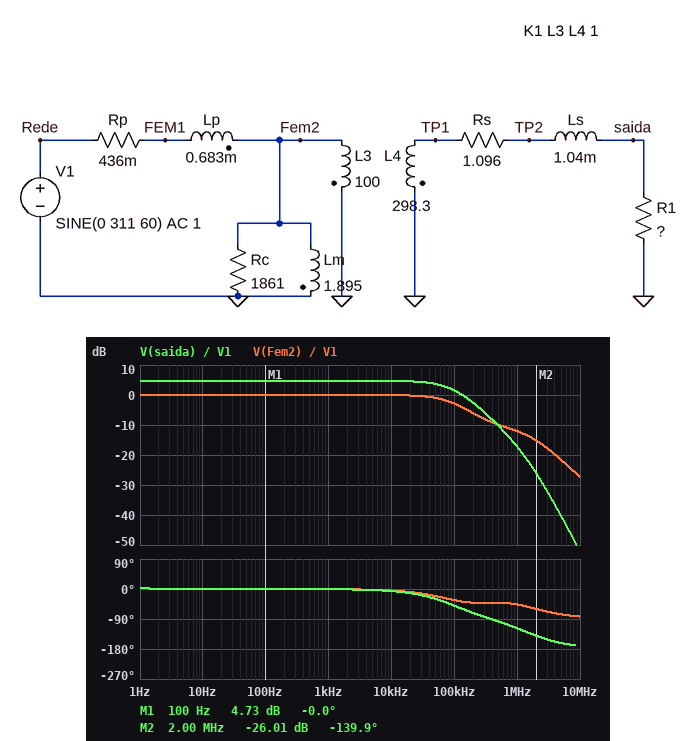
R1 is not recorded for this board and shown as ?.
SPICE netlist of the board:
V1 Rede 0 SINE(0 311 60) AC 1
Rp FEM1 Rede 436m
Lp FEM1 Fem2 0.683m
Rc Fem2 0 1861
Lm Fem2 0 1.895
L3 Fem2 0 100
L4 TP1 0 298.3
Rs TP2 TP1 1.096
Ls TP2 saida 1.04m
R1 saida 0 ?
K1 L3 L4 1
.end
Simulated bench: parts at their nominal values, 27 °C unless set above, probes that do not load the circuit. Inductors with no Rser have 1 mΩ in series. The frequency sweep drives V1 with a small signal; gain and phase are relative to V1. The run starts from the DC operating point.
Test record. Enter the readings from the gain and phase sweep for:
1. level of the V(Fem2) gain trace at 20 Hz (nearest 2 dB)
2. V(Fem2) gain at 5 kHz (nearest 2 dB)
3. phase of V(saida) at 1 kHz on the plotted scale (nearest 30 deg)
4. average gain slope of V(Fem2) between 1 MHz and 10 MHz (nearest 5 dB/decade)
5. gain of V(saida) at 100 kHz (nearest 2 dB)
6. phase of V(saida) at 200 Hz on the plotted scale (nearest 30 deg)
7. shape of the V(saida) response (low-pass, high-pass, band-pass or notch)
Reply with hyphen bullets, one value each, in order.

- 0 dB
- 0 dB
- 0 deg
- -15 dB/decade
- 2 dB
- 0 deg
- low-pass
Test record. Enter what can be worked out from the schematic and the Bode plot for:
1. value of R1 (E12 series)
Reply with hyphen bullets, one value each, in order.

- 2.2 kΩ
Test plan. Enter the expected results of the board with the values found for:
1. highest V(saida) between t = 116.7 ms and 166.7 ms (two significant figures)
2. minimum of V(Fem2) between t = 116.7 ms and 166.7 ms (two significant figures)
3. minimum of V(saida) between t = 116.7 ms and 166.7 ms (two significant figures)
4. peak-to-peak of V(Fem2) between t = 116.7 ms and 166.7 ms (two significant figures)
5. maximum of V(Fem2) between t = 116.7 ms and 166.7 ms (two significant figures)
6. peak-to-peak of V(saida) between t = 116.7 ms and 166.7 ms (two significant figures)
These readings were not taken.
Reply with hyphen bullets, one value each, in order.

- 540 V
- -310 V
- -540 V
- 620 V
- 310 V
- 1.1 kV
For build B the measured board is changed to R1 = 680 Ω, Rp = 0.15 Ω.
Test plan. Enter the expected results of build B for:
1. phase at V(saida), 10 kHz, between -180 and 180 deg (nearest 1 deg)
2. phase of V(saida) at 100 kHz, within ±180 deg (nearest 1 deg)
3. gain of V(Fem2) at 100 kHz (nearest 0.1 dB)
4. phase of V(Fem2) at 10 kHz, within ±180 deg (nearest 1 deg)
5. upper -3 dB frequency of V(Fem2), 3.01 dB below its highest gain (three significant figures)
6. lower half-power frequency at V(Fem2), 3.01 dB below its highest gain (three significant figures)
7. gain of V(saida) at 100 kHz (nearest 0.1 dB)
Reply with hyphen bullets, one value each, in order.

- -17 deg
- -76 deg
- -7.2 dB
- -12 deg
- 37.5 kHz
- 13.0 mHz
- -5.3 dB
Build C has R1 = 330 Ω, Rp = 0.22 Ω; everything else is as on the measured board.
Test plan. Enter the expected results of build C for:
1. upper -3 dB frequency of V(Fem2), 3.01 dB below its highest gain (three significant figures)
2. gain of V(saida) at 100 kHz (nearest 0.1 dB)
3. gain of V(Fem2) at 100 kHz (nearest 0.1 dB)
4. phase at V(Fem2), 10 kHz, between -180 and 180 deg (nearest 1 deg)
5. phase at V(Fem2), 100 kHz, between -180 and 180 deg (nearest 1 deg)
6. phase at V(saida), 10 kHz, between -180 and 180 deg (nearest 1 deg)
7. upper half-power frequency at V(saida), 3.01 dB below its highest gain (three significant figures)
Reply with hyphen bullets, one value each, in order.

- 18.9 kHz
- -11.0 dB
- -8.8 dB
- -20 deg
- -22 deg
- -31 deg
- 16.7 kHz
